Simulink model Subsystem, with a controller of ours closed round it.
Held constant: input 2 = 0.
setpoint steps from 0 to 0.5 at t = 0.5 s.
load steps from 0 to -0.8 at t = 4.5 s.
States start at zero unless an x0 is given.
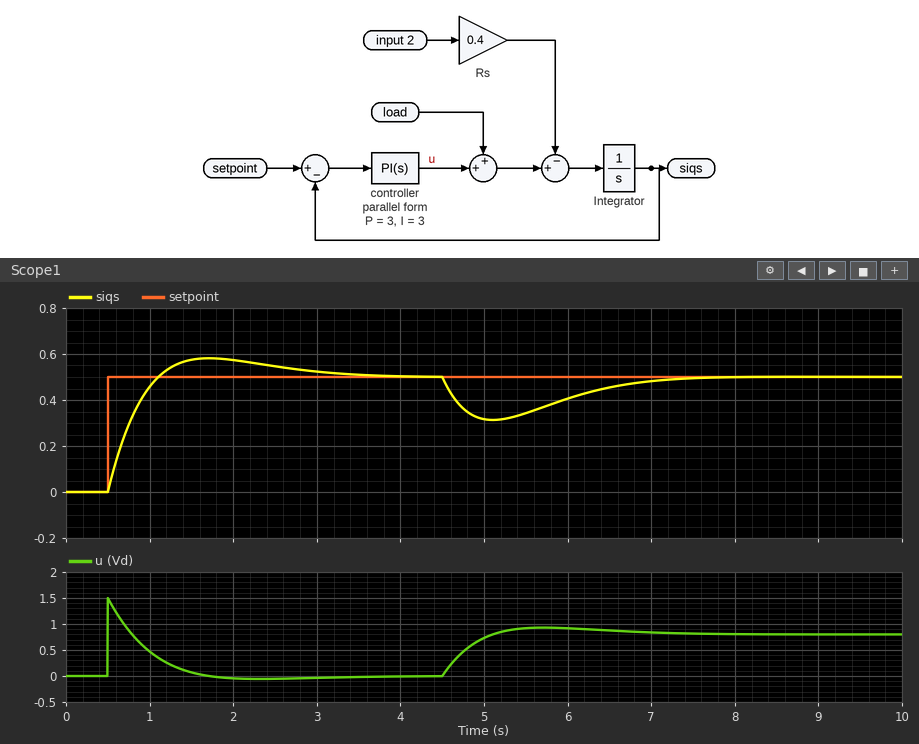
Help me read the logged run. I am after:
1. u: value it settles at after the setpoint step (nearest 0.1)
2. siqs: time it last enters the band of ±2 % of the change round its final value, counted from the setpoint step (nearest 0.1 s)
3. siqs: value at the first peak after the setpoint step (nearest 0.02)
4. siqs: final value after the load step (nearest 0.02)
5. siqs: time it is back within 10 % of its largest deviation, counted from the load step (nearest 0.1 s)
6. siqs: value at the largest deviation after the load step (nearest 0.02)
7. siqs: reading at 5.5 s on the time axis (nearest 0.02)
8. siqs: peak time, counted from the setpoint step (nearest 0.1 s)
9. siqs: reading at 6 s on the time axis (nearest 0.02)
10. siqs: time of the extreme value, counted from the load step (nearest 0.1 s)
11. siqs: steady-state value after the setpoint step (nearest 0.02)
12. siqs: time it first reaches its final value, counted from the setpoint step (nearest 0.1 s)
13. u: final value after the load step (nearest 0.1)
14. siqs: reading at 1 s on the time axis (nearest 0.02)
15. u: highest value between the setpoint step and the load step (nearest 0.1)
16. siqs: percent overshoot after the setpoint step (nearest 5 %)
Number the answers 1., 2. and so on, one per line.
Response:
1. 0.0
2. 3.0 s
3. 0.58
4. 0.50
5. 2.5 s
6. 0.32
7. 0.34
8. 1.2 s
9. 0.40
10. 0.6 s
11. 0.50
12. 0.6 s
13. 0.8
14. 0.46
15. 1.5
16. 15 %
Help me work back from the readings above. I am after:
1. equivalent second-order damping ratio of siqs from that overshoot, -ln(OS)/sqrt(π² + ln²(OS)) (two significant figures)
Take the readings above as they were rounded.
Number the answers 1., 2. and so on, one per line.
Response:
1. 0.52
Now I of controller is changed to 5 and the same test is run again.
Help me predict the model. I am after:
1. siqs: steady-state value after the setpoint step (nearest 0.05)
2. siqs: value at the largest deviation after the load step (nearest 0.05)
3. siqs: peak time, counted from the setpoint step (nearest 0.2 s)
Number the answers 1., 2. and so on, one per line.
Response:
1. 0.50
2. 0.35
3. 1.0 s
